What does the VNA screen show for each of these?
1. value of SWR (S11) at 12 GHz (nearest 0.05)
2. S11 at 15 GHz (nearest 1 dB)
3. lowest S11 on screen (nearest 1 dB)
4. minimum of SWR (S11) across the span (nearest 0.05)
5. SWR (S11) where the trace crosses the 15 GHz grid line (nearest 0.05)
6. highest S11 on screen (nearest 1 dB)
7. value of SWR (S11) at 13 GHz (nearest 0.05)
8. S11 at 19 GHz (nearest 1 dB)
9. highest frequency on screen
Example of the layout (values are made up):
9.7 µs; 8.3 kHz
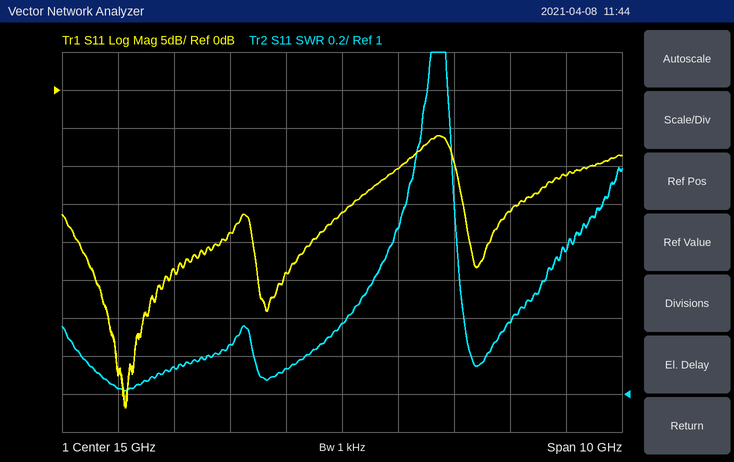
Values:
1.15; -16 dB; -42 dB; 1.00; 1.35; -6 dB; 1.25; -11 dB; 20 GHz
